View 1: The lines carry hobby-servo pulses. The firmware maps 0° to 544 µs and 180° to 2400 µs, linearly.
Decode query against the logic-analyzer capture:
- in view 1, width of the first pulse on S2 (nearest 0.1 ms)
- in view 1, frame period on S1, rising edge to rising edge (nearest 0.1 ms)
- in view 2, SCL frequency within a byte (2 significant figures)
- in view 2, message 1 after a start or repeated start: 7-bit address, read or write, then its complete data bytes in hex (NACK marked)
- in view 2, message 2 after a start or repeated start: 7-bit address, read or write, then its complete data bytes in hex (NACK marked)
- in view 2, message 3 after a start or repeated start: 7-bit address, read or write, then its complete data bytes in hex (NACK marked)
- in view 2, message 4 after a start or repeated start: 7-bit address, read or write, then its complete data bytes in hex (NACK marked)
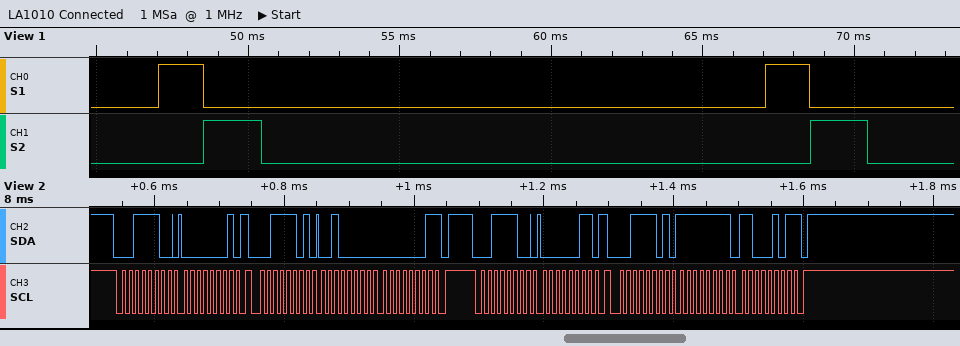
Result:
1.9 ms
20.0 ms
100 kHz
0x1E write: 01
0x1E read: 20 01 NACK
0x1E write: 03
0x1E read: FF C5 NACK
